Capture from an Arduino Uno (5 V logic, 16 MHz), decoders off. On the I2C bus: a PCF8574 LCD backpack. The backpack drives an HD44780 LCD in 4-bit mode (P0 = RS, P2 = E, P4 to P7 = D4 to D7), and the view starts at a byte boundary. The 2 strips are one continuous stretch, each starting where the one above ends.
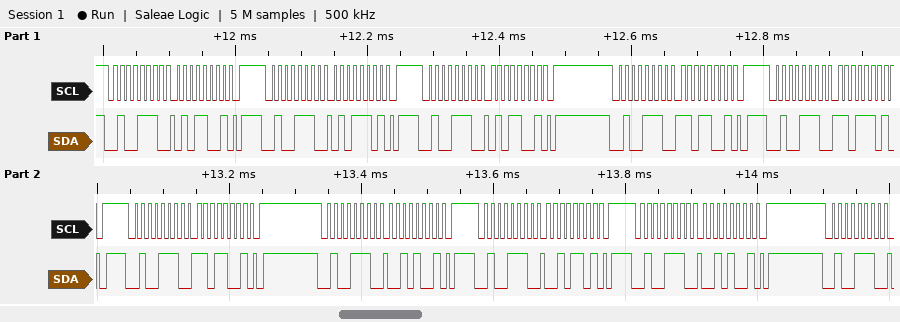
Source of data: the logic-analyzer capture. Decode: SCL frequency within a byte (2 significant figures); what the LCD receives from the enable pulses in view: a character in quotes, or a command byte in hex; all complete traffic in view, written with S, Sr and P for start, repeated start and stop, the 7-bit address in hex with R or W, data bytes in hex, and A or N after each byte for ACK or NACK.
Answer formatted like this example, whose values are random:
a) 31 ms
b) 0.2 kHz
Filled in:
a) 100 kHz
b) ']'
c) S 27W A 59 A P S 27W A 5D A P S 27W A 59 A P S 27W A D9 A P S 27W A DD A P S 27W A D9 A P S 27W A 29 A P S 27W A 2D A P S 27W A 29 A P S 27W A
